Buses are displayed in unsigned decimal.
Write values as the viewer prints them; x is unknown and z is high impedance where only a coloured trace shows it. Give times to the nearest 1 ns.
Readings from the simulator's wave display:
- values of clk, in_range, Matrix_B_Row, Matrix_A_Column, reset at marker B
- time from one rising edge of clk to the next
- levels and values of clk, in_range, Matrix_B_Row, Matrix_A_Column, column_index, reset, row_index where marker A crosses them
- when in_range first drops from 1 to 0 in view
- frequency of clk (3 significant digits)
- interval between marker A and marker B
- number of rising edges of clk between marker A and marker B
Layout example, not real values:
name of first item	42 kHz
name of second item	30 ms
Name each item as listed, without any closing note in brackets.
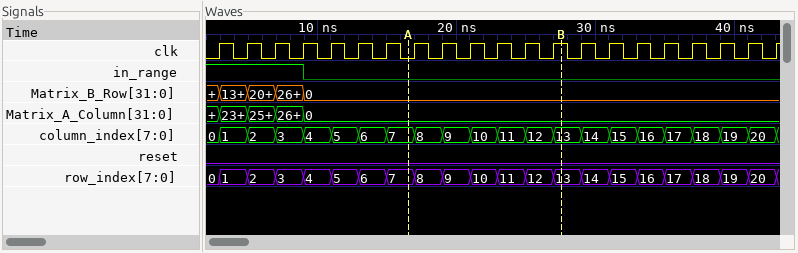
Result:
values of clk, in_range, Matrix_B_Row, Matrix_A_Column, reset at marker B	clk=1, in_range=0, Matrix_B_Row=0, Matrix_A_Column=0, reset=0
time from one rising edge of clk to the next	2 ns
levels and values of clk, in_range, Matrix_B_Row, Matrix_A_Column, column_index, reset, row_index where marker A crosses them	clk=0, in_range=0, Matrix_B_Row=0, Matrix_A_Column=0, column_index=7, reset=0, row_index=7
when in_range first drops from 1 to 0 in view	9 ns
frequency of clk	500 MHz
interval between marker A and marker B	11 ns
number of rising edges of clk between marker A and marker B	6
